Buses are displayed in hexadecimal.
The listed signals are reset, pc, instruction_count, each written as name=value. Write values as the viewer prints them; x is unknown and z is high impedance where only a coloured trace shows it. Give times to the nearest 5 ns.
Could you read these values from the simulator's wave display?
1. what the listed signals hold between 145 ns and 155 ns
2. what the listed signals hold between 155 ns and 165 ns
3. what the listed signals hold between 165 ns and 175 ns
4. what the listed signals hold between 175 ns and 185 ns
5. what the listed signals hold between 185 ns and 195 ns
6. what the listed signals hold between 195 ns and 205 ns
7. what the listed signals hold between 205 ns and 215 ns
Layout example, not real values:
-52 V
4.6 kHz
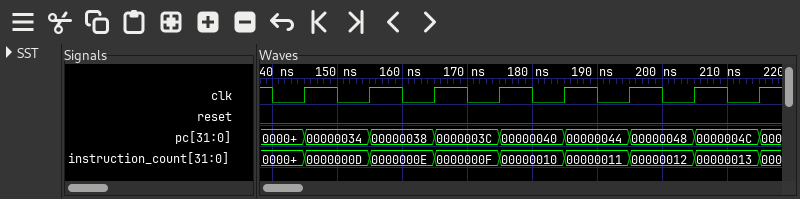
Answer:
reset=0, pc=00000034, instruction_count=0000000D
reset=0, pc=00000038, instruction_count=0000000E
reset=0, pc=0000003C, instruction_count=0000000F
reset=0, pc=00000040, instruction_count=00000010
reset=0, pc=00000044, instruction_count=00000011
reset=0, pc=00000048, instruction_count=00000012
reset=0, pc=0000004C, instruction_count=00000013
